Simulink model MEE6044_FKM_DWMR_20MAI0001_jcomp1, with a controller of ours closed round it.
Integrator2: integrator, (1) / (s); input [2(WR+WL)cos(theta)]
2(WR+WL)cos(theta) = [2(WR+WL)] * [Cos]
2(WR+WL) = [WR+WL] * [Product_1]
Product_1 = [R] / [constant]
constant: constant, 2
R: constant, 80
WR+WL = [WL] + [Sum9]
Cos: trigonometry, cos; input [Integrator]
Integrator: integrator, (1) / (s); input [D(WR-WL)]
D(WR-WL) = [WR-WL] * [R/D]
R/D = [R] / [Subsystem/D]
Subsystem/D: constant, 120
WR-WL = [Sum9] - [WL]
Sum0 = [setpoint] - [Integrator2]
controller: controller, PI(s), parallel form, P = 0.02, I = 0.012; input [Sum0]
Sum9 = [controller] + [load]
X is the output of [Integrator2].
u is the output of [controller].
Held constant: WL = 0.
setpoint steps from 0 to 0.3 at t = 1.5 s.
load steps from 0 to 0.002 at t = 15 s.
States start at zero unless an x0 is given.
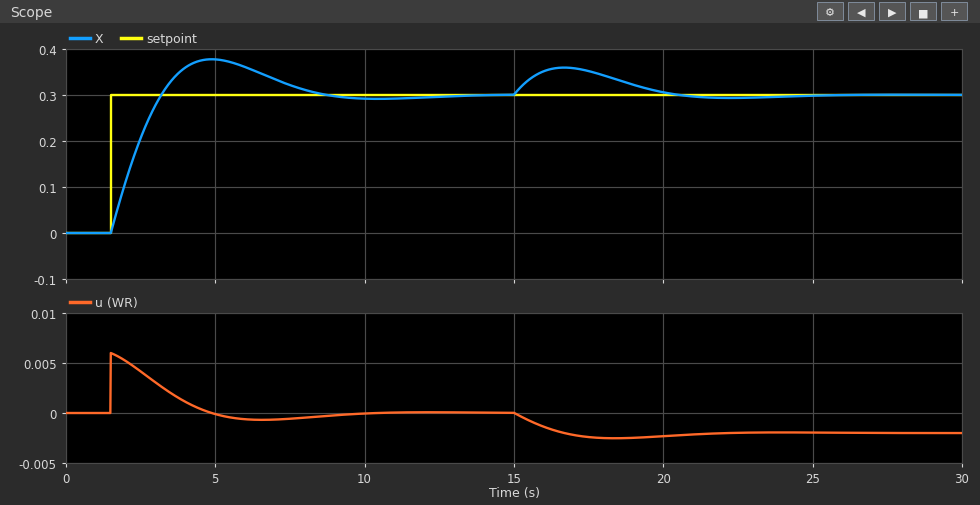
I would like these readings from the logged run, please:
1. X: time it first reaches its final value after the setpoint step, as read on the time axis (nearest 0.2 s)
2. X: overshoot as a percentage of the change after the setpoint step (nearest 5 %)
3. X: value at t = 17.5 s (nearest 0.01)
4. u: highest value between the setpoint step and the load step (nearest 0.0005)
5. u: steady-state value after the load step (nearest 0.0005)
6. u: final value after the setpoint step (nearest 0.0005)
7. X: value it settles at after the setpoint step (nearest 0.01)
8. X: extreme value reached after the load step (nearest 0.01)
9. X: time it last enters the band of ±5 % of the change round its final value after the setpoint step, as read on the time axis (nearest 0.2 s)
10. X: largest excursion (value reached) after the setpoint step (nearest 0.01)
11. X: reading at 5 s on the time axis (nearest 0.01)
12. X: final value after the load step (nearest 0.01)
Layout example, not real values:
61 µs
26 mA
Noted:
3.2 s
25 %
0.35
0.0060
-0.0020
0.0000
0.30
0.36
7.8 s
0.38
0.38
0.30
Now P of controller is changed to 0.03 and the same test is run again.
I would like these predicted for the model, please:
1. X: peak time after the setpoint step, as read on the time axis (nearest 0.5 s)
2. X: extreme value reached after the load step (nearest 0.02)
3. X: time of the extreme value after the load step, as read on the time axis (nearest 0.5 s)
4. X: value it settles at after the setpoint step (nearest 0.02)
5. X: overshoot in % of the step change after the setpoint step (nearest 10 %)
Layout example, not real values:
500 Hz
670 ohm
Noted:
4.5 s
0.34
16.5 s
0.30
20 %
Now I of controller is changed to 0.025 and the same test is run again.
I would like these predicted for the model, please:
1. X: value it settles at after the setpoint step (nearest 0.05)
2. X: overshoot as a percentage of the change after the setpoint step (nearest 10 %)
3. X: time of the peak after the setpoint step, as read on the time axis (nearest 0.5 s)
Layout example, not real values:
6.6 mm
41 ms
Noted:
0.30
40 %
4.0 s
